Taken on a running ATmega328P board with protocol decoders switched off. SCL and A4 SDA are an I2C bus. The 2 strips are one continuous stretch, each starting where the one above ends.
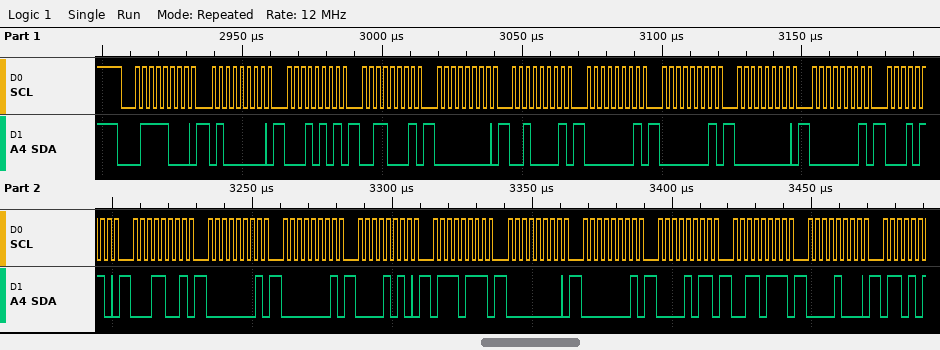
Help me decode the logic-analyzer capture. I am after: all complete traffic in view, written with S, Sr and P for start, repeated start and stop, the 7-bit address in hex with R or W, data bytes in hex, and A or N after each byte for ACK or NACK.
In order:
S 3CW A 40 A 15 A 31 A 00 A 21 A 01 A 01 A 00 A 01 A 16 A 19 A 01 A 01 A 0A A 77 A 00 A 01 A 0B A 37 A 08 A
